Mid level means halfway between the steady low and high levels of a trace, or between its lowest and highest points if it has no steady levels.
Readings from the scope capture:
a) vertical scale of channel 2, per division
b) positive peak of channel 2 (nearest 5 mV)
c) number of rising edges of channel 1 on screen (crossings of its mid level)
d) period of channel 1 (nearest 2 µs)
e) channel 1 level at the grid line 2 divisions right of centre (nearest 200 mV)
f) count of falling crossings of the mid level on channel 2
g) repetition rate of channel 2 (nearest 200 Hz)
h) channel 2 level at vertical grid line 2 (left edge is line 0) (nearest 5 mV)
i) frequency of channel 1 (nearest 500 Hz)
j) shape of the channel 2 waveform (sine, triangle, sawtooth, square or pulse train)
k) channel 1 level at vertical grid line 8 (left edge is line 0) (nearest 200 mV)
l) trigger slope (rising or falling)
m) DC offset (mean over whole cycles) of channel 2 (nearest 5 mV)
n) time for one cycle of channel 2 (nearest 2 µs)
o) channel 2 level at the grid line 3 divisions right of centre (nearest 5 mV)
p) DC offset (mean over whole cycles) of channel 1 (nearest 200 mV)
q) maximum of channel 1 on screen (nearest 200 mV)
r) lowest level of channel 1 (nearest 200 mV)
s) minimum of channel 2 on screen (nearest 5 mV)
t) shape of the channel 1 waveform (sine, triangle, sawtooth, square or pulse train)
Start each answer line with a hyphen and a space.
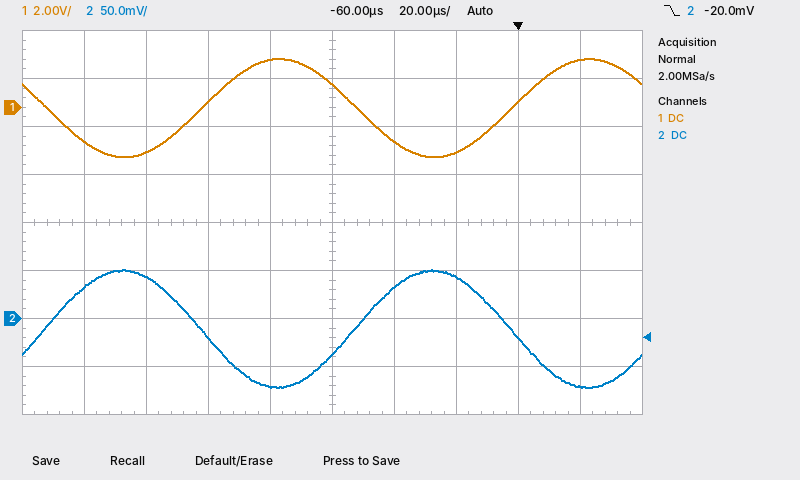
- 50 mV
- 50 mV
- 2
- 100 µs
- -1.8 V
- 2
- 10.0 kHz
- 45 mV
- 10.0 kHz
- sine
- 200 mV
- falling
- -10 mV
- 100 µs
- -20 mV
- 0.0 V
- 2.0 V
- -2.0 V
- -70 mV
- sine
